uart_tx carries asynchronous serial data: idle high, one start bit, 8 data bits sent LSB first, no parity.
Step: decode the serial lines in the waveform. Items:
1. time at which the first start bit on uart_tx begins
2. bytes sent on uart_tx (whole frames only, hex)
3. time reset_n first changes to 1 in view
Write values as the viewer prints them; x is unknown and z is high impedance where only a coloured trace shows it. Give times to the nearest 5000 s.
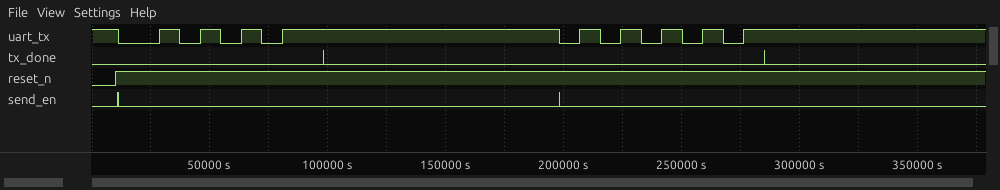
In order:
10000 s
AA, 55
10000 s
